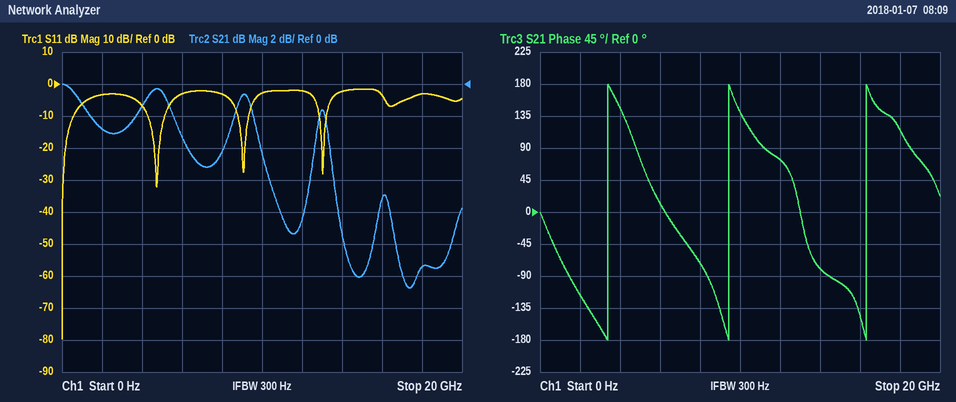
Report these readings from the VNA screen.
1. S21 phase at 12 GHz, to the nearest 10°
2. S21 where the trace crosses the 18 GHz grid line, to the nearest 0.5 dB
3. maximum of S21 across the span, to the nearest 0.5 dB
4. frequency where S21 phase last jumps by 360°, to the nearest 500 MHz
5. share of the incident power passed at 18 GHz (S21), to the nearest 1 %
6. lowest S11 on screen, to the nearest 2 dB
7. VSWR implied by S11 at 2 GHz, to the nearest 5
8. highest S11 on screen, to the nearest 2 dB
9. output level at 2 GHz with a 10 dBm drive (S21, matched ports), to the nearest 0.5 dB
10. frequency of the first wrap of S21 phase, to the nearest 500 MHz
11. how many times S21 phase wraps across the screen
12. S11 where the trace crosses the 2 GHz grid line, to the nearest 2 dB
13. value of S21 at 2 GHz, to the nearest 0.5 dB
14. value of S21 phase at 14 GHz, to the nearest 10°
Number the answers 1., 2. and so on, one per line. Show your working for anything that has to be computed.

1. 70°
2. -11.5 dB
3. 0.0 dB
4. 16.5 GHz
5. 10^(-11.5/10) ≈ 7 %
6. -80 dB
7. |Γ| = 10^(-4/20) = 0.6310; VSWR = (1 + 0.6310)/(1 − 0.6310) ≈ 4.42, so 5 to the nearest 5
8. -2 dB
9. 10 dBm + (-3.0 dB) = 7.0 dBm
10. 3.5 GHz
11. 3
12. -4 dB
13. -3.0 dB
14. -80°
